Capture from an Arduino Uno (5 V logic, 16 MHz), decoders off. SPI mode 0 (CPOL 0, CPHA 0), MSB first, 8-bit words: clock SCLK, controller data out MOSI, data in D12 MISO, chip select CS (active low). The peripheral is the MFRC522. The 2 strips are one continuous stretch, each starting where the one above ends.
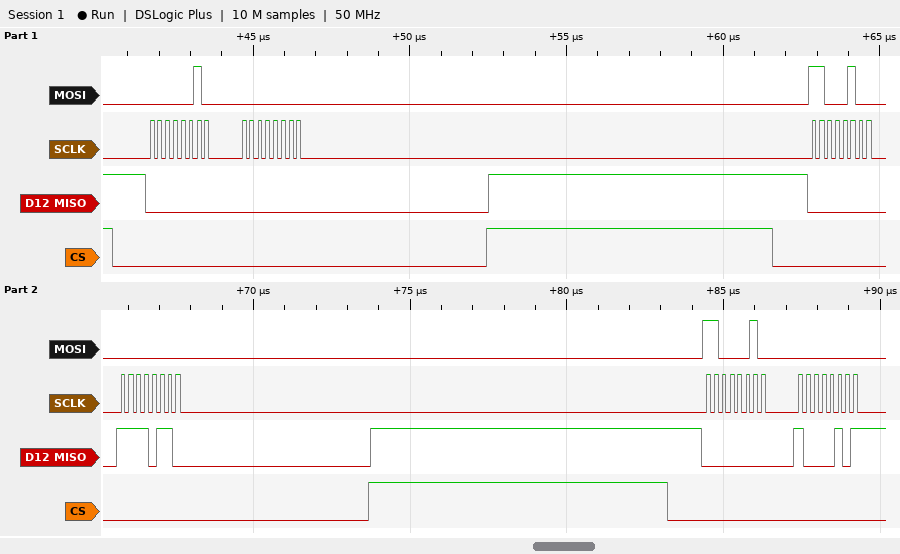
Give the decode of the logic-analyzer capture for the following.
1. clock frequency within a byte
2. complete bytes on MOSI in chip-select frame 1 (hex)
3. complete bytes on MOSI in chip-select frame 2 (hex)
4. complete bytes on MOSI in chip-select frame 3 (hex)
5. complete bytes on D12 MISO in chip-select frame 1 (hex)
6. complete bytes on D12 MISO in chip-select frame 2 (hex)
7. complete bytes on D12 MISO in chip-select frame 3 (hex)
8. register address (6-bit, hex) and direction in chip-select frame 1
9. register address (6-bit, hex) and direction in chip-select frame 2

4 MHz
02 00
C4 00
C2 00
00 00
00 F6
00 85
0x01 write
0x22 read
